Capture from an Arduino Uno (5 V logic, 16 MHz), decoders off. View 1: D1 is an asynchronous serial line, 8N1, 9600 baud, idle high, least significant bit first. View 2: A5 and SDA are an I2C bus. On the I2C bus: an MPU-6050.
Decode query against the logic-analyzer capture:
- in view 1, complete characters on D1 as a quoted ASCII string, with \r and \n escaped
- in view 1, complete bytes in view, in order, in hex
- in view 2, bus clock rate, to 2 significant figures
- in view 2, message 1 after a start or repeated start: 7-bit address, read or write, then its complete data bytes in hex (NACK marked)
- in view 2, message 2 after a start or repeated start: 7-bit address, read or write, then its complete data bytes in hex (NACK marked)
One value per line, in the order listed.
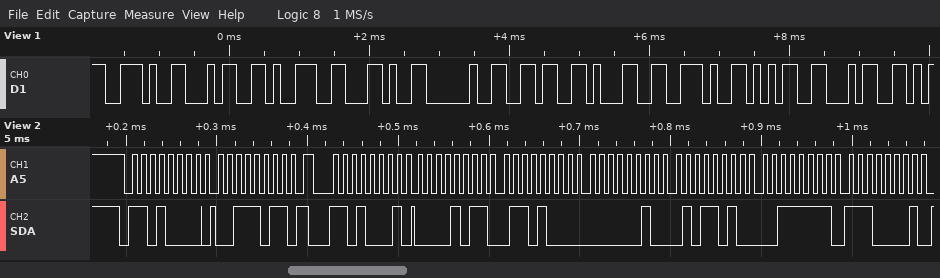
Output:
".49, 61.54"
0x2E 0x34 0x39 0x2C 0x20 0x36 0x31 0x2E 0x35 0x34
100 kHz
0x68 write: 3B
0x68 read: 0B 68 02 5A 3F E1
